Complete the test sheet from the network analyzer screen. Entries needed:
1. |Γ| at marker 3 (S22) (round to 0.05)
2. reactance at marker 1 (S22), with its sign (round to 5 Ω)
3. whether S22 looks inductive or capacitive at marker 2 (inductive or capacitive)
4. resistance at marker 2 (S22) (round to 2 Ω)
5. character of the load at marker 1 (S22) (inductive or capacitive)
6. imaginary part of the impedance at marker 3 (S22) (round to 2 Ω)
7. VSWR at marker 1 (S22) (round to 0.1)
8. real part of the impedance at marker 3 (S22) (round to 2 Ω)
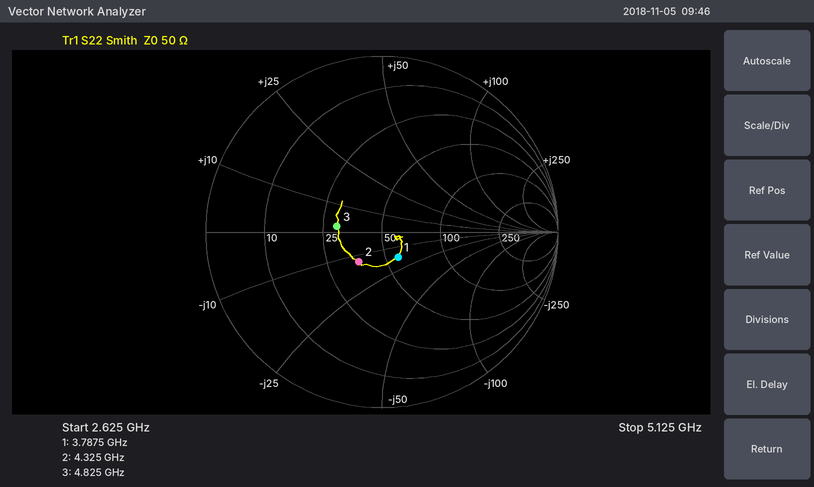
0.25
-15 Ω
capacitive
36 Ω
capacitive
+2 Ω
1.4
30 Ω
